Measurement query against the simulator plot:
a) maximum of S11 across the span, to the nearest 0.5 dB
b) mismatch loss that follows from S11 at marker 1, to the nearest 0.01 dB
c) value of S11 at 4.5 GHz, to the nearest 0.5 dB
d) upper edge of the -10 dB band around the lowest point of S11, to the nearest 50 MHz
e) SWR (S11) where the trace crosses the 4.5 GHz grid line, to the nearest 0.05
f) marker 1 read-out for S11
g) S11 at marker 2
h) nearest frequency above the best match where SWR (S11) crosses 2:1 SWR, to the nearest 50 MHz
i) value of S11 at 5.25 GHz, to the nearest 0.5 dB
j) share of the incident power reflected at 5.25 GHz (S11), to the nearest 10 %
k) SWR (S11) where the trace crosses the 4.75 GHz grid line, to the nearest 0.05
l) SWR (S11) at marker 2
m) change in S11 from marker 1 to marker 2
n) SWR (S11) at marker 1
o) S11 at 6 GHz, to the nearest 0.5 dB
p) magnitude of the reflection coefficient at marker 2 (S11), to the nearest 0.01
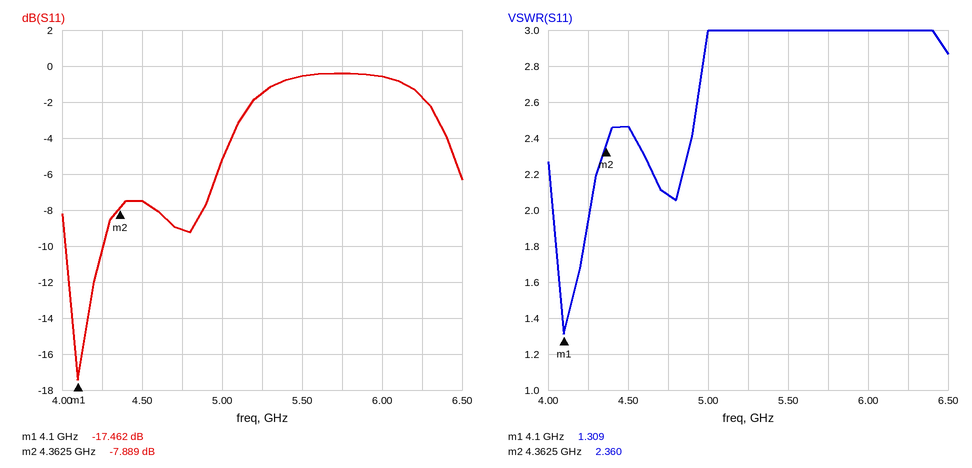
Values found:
-0.5 dB
0.08 dB
-7.5 dB
4.25 GHz
2.45
-17.462 dB
-7.889 dB
4.25 GHz
-1.5 dB
70 %
2.10
2.360
9.573 dB
1.309
-0.5 dB
0.40
